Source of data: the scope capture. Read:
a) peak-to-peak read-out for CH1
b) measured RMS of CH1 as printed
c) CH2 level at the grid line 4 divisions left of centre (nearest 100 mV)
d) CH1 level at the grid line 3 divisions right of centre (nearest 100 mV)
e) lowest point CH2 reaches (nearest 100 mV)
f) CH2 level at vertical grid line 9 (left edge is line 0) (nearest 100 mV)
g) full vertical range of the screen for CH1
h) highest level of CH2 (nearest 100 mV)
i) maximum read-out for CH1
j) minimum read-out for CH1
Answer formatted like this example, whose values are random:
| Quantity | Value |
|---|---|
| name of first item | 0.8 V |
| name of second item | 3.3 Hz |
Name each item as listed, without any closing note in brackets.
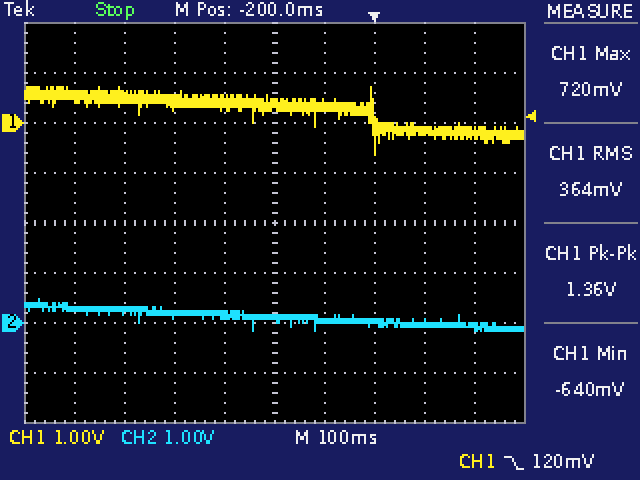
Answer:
| Quantity | Value |
|---|---|
| peak-to-peak read-out for CH1 | 1.36 V |
| measured RMS of CH1 as printed | 364 mV |
| CH2 level at the grid line 4 divisions left of centre | 300 mV |
| CH1 level at the grid line 3 divisions right of centre | -200 mV |
| lowest point CH2 reaches | -200 mV |
| CH2 level at vertical grid line 9 (left edge is line 0) | -100 mV |
| full vertical range of the screen for CH1 | 8 V |
| highest level of CH2 | 500 mV |
| maximum read-out for CH1 | 720 mV |
| minimum read-out for CH1 | -640 mV |
